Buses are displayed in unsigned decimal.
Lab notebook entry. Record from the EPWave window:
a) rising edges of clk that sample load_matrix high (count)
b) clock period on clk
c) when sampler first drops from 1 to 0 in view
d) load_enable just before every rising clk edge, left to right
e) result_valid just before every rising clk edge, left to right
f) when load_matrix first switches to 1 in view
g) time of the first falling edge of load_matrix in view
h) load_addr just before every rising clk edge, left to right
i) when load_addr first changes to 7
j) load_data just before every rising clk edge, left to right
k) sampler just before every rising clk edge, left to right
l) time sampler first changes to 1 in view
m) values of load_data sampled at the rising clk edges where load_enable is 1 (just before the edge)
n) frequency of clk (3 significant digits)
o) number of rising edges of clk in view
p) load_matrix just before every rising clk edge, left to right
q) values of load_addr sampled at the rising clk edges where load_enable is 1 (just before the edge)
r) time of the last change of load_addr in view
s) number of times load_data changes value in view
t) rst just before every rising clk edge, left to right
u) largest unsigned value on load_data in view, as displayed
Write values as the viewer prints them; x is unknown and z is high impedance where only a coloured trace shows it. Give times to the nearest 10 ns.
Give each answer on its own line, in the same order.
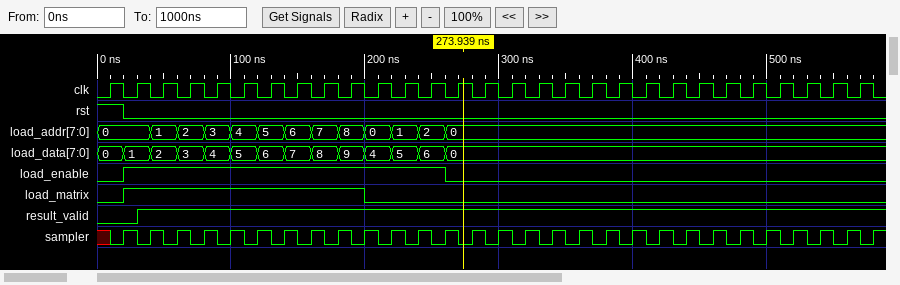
9
20 ns
30 ns
0 1 1 1 1 1 1 1 1 1 1 1 1 0 0 0 0 0 0 0 0 0 0 0 0 0 0 0 0
0 0 1 1 1 1 1 1 1 1 1 1 1 1 1 1 1 1 1 1 1 1 1 1 1 1 1 1 1
20 ns
200 ns
0, 0, 1, 2, 3, 4, 5, 6, 7, 8, 0, 1, 2, 0, 0, 0, 0, 0, 0, 0, 0, 0, 0, 0, 0, 0, 0, 0, 0
160 ns
0, 1, 2, 3, 4, 5, 6, 7, 8, 9, 4, 5, 6, 0, 0, 0, 0, 0, 0, 0, 0, 0, 0, 0, 0, 0, 0, 0, 0
x 1 1 1 1 1 1 1 1 1 1 1 1 1 1 1 1 1 1 1 1 1 1 1 1 1 1 1 1
20 ns
1, 2, 3, 4, 5, 6, 7, 8, 9, 4, 5, 6
50.0 MHz
29
0 1 1 1 1 1 1 1 1 1 0 0 0 0 0 0 0 0 0 0 0 0 0 0 0 0 0 0 0
0, 1, 2, 3, 4, 5, 6, 7, 8, 0, 1, 2
260 ns
13
1 0 0 0 0 0 0 0 0 0 0 0 0 0 0 0 0 0 0 0 0 0 0 0 0 0 0 0 0
9
